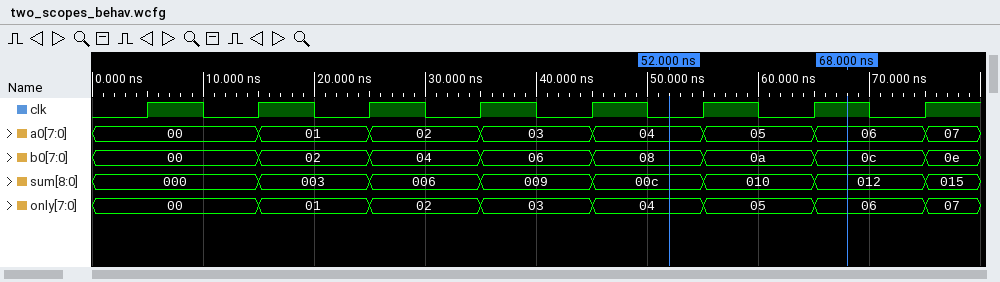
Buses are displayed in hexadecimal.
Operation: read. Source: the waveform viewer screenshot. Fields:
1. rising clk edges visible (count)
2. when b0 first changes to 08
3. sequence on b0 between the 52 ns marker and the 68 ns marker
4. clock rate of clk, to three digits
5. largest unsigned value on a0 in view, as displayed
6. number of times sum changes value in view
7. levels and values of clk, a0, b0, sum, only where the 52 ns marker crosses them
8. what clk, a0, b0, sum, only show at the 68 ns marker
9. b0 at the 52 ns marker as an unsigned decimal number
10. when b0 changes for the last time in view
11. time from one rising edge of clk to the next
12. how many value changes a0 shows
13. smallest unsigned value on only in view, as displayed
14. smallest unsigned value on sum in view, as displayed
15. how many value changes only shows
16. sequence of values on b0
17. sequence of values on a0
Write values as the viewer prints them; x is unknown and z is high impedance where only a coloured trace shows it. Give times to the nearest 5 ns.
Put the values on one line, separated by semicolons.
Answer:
8; 45 ns; 08, 0a, 0c; 100 MHz; 07; 7; clk=0, a0=04, b0=08, sum=00c, only=04; clk=1, a0=06, b0=0c, sum=012, only=06; 8; 75 ns; 10 ns; 7; 00; 000; 7; 00, 02, 04, 06, 08, 0a, 0c, 0e; 00, 01, 02, 03, 04, 05, 06, 07
